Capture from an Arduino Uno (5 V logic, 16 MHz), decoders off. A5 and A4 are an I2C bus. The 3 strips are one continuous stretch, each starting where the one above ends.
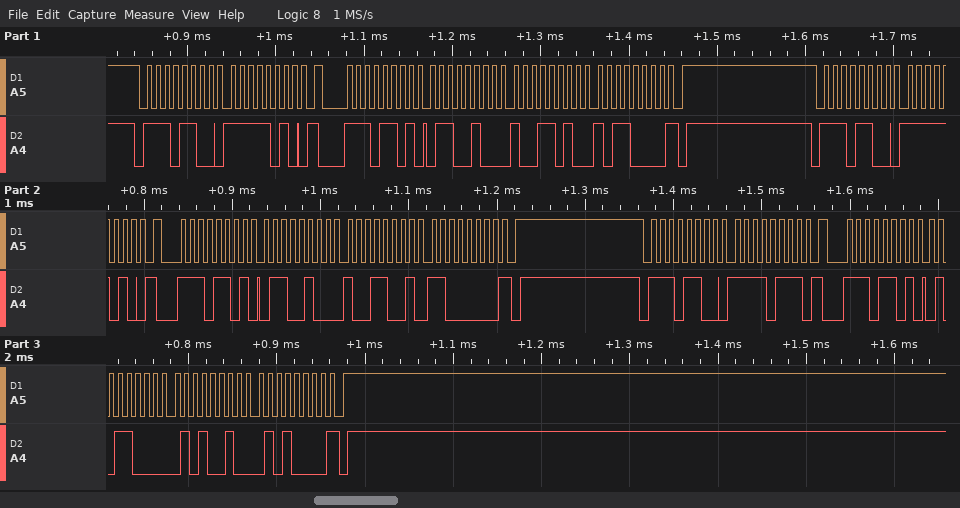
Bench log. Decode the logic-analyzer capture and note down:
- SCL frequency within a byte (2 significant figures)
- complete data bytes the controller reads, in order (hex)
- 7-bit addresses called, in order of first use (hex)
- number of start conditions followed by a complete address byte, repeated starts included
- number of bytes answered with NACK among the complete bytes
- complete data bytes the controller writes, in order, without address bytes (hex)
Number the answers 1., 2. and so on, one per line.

1. 100 kHz
2. 64 9A B0 64 99 C0 58 52 50
3. 0x76
4. 6
5. 3
6. FA FA F7
